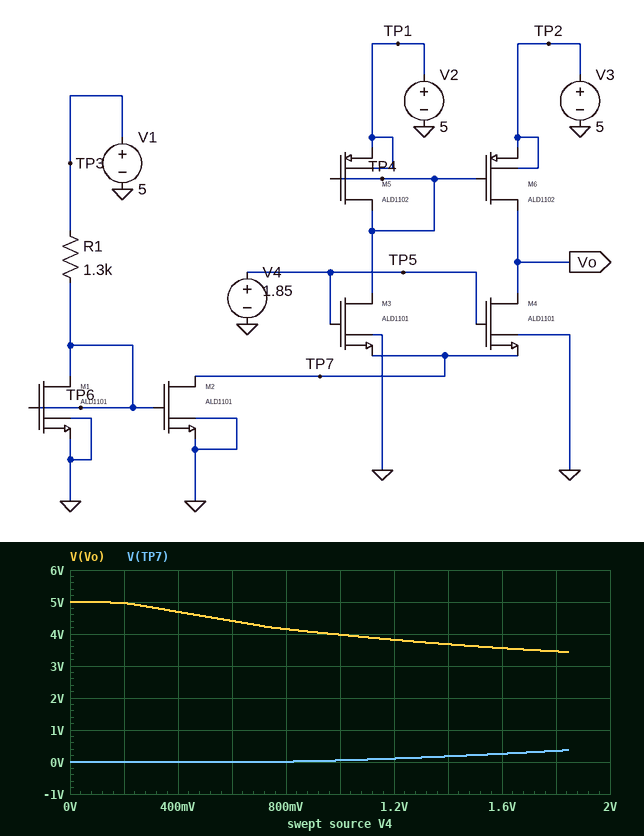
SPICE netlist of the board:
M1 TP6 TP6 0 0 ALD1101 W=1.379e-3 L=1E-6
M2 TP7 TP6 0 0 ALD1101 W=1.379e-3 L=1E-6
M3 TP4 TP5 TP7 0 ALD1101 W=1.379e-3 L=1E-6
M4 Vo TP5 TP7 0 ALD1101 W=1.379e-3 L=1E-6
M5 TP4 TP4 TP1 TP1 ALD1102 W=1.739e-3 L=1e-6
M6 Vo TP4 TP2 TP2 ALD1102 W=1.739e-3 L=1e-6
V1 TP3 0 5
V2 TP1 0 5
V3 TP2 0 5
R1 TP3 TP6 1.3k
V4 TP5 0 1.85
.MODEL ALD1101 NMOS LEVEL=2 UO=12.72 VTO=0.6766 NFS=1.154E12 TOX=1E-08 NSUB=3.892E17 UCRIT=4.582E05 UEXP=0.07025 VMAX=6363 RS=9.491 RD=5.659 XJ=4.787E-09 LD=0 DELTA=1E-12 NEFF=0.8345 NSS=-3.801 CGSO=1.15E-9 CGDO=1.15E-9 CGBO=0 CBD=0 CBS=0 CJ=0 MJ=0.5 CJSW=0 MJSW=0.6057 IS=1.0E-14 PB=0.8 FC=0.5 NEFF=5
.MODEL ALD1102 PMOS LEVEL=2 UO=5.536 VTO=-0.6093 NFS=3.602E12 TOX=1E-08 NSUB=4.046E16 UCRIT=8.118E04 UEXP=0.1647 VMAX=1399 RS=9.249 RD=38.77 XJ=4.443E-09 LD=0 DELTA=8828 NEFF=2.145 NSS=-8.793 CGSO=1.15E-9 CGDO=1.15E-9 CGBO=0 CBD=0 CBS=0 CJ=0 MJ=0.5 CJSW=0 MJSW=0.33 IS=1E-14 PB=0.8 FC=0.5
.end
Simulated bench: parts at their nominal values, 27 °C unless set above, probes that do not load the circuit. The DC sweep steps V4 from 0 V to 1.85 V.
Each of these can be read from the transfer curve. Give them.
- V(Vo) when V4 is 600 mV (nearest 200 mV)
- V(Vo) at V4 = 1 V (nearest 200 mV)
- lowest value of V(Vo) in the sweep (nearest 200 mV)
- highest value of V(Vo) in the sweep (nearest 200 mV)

4.4 V
4.0 V
3.4 V
5.0 V
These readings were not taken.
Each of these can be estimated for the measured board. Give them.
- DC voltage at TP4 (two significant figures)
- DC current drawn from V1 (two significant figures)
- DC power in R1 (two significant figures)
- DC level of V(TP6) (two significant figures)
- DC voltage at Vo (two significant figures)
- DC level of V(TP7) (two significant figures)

3.4 V
2.5 mA
8.0 mW
1.8 V
3.4 V
370 mV
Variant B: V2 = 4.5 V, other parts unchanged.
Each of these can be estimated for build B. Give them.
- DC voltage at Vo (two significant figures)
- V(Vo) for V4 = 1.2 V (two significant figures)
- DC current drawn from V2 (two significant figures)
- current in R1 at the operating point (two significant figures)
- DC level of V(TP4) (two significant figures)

4.7 V
4.9 V
870 µA
2.5 mA
2.9 V
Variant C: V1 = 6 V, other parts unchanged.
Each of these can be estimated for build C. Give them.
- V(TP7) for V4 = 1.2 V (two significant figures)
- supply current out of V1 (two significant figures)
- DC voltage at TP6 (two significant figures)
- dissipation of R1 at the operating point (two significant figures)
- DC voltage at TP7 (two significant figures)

100 mV
3.1 mA
1.9 V
13 mW
350 mV
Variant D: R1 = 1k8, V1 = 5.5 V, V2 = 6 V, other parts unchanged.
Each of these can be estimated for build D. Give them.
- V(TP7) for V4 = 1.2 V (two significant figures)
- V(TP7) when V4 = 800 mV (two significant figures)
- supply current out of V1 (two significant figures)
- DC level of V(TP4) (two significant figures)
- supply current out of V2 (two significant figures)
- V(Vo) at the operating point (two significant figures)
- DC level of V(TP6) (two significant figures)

73 mV
6.9 mV
2.1 mA
4.2 V
1.3 mA
280 mV
1.7 V
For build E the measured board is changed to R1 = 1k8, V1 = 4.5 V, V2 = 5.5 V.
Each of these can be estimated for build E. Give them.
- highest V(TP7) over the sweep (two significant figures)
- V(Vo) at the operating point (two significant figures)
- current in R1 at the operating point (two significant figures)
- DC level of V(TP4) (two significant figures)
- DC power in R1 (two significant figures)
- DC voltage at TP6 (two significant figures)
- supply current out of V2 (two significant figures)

350 mV
430 mV
1.6 mA
3.9 V
4.8 mW
1.6 V
980 µA
